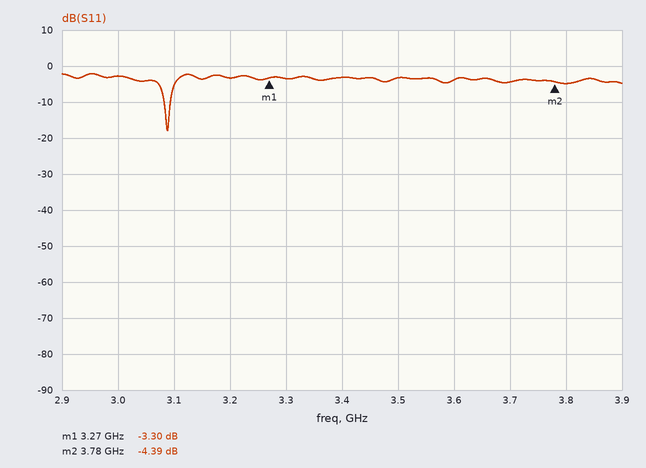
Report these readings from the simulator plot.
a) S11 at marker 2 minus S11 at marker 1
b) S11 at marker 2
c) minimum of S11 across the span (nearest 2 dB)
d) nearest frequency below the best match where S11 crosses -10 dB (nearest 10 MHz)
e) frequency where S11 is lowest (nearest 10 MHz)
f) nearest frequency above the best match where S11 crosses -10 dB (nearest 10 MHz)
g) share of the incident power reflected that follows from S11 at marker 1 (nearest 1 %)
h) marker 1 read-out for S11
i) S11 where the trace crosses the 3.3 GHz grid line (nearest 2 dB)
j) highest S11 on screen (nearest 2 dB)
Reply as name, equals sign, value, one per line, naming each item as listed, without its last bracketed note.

S11 at marker 2 minus S11 at marker 1 = -1.09 dB
S11 at marker 2 = -4.39 dB
minimum of S11 across the span = -18 dB
nearest frequency below the best match where S11 crosses -10 dB = 3.08 GHz
frequency where S11 is lowest = 3.09 GHz
nearest frequency above the best match where S11 crosses -10 dB = 3.09 GHz
share of the incident power reflected that follows from S11 at marker 1 = 47 %
marker 1 read-out for S11 = -3.30 dB
S11 where the trace crosses the 3.3 GHz grid line = -4 dB
highest S11 on screen = -2 dB
